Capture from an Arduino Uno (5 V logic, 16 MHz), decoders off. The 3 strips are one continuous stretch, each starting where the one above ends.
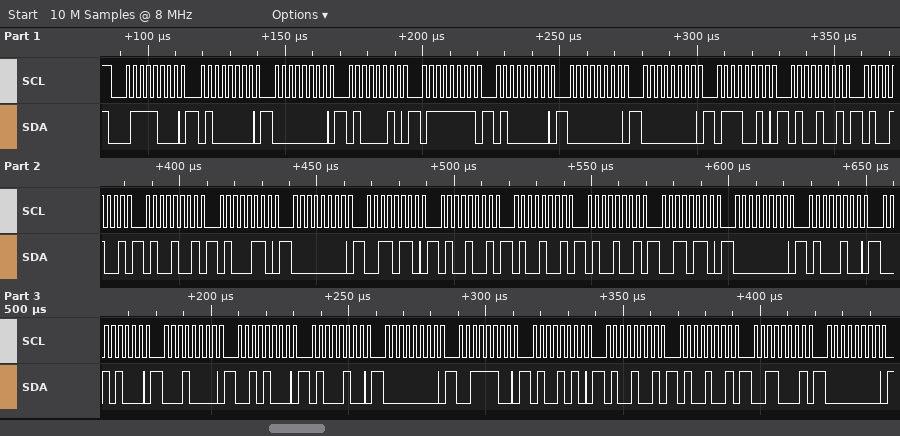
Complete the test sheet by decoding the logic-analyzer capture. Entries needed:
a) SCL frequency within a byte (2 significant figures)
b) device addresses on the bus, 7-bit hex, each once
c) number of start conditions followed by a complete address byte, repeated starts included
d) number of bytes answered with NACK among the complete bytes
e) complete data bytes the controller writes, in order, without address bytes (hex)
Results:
400 kHz
0x3C
1
0
40 00 42 7F 40 00 00 72 49 49 49 46 00 36 49 49 49 36 00 44 28 10 28 44 00 3C 4A 49 49 31 00
